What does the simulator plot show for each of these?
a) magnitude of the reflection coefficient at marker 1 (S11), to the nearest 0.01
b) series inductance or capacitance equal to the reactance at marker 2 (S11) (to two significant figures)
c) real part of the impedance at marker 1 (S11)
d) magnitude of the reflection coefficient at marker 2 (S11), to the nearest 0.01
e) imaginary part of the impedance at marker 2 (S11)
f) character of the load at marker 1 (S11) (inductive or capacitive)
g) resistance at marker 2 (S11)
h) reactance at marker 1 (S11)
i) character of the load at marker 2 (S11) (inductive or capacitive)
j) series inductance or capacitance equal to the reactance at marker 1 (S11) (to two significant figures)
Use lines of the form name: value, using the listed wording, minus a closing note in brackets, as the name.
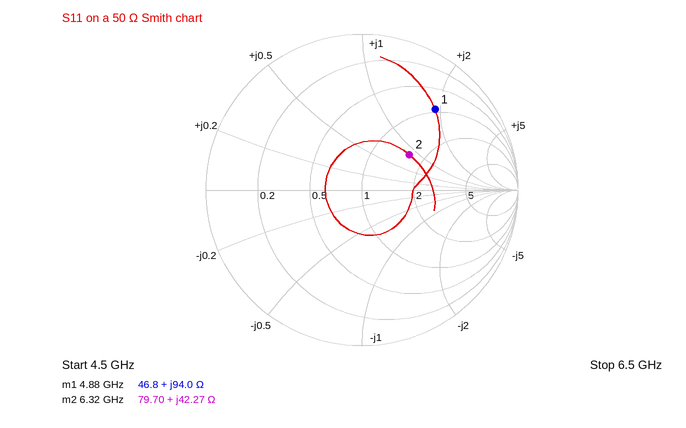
magnitude of the reflection coefficient at marker 1 (S11), to the nearest 0.01: 0.70
series inductance or capacitance equal to the reactance at marker 2 (S11): 1.1 nH
real part of the impedance at marker 1: 46.8 Ω
magnitude of the reflection coefficient at marker 2 (S11), to the nearest 0.01: 0.38
imaginary part of the impedance at marker 2: +42.27 Ω
character of the load at marker 1 (S11): inductive
resistance at marker 2: 79.70 Ω
reactance at marker 1: +94.0 Ω
character of the load at marker 2 (S11): inductive
series inductance or capacitance equal to the reactance at marker 1 (S11): 3.1 nH
